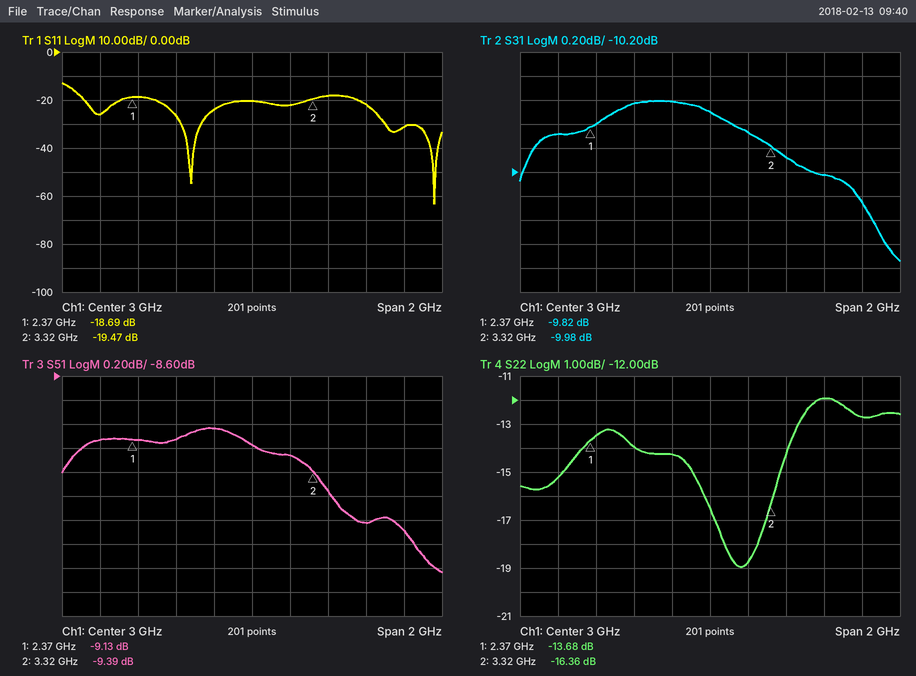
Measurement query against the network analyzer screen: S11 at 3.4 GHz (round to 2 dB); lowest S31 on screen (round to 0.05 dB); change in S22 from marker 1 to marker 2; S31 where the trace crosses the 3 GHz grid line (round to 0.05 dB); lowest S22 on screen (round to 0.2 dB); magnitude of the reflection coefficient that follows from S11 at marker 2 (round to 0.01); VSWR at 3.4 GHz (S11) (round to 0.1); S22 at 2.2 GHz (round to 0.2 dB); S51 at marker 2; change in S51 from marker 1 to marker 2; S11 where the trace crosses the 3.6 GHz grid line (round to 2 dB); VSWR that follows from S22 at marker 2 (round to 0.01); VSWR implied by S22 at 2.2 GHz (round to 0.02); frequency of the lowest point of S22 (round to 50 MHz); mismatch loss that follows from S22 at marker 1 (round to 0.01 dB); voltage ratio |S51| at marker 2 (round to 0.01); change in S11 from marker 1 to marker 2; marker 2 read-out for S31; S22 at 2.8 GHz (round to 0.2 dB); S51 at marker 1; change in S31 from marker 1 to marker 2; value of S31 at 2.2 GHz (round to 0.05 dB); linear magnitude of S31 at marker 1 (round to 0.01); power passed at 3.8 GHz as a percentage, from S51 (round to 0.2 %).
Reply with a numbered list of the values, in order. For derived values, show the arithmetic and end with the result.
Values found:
1. -18 dB
2. -10.95 dB
3. -16.36 − (-13.68) = -2.68 dB
4. -9.70 dB
5. -19.0 dB
6. 10^(-19.47/20) ≈ 0.11
7. |Γ| = 10^(-18/20) = 0.1259; VSWR = (1 + 0.1259)/(1 − 0.1259) ≈ 1.3
8. -15.2 dB
9. -9.39 dB
10. -9.39 − (-9.13) = -0.26 dB
11. -22 dB
12. (1 + 0.1521)/(1 − 0.1521) ≈ 1.36
13. |Γ| = 10^(-15.2/20) = 0.1738; VSWR = (1 + 0.1738)/(1 − 0.1738) ≈ 1.42
14. 3.15 GHz
15. −10 log10(1 − 10^(-13.68/10)) ≈ 0.19 dB
16. 10^(-9.39/20) ≈ 0.34
17. -19.47 − (-18.69) = -0.78 dB
18. -9.98 dB
19. -14.2 dB
20. -9.13 dB
21. -9.98 − (-9.82) = -0.16 dB
22. -9.90 dB
23. 10^(-9.82/20) ≈ 0.32
24. 10^(-9.9/10) ≈ 10.2 %
